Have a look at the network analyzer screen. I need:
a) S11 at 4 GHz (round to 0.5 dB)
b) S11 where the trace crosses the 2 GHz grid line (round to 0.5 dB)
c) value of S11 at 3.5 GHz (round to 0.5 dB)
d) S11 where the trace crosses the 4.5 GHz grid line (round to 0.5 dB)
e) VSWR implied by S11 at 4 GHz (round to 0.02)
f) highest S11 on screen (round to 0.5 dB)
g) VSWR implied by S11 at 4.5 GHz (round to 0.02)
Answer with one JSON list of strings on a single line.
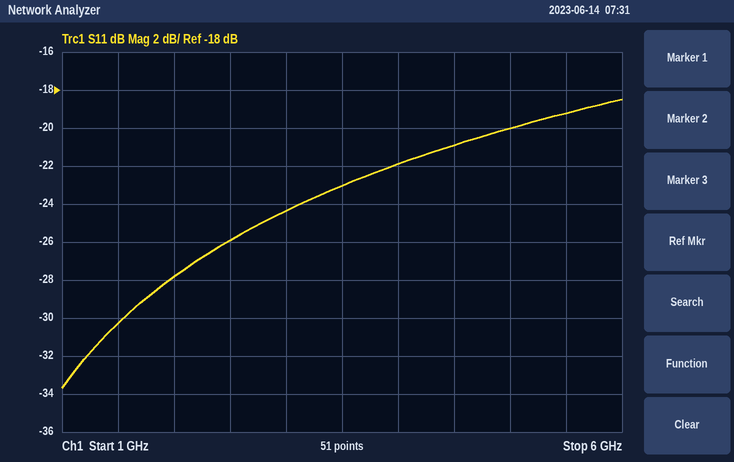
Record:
["-22.0 dB", "-28.0 dB", "-23.0 dB", "-21.0 dB", "1.18", "-18.5 dB", "1.20"]
